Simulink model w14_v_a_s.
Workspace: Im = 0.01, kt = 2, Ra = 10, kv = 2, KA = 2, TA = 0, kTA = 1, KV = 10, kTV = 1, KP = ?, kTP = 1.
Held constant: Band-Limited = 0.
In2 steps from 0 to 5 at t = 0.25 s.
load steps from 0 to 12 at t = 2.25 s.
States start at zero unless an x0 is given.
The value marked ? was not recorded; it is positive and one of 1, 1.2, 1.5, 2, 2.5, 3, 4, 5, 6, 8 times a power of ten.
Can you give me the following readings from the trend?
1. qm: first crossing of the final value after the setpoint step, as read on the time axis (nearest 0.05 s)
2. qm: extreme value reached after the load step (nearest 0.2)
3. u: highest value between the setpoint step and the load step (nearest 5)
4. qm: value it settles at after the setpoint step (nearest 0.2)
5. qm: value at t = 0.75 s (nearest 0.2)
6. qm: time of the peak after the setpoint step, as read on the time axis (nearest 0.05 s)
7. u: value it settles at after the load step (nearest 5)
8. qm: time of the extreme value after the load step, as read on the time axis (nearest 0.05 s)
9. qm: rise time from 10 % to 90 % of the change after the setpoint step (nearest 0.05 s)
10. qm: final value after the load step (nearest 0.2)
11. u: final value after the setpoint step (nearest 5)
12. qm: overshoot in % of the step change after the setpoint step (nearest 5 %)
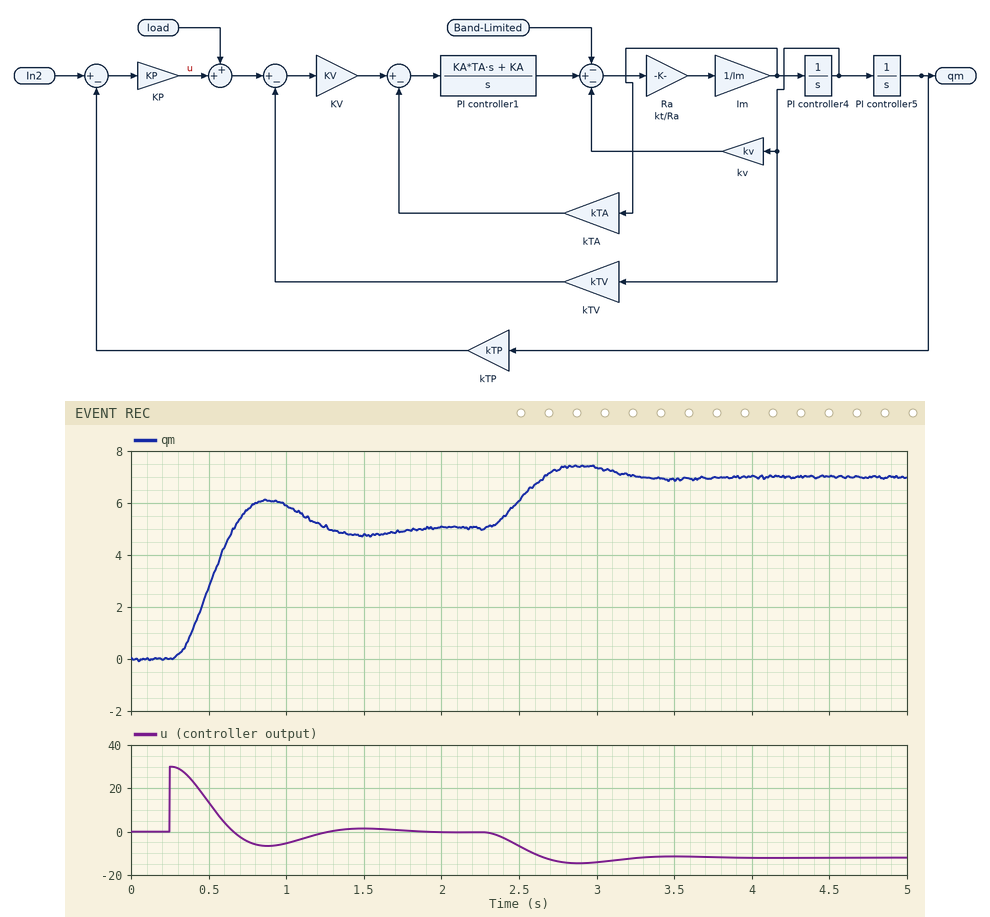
0.65 s
7.4
30
5.0
5.8
0.90 s
-10
2.90 s
0.25 s
7.0
0
20 %
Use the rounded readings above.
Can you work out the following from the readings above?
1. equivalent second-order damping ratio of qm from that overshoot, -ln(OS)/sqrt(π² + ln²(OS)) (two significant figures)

0.46
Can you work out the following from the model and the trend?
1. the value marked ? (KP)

6
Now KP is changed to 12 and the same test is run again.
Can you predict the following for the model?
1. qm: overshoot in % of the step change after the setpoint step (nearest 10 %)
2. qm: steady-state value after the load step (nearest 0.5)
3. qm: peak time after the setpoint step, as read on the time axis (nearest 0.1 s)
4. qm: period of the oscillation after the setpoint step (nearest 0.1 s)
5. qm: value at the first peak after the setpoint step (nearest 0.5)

40 %
6.0
0.7 s
0.8 s
7.0
